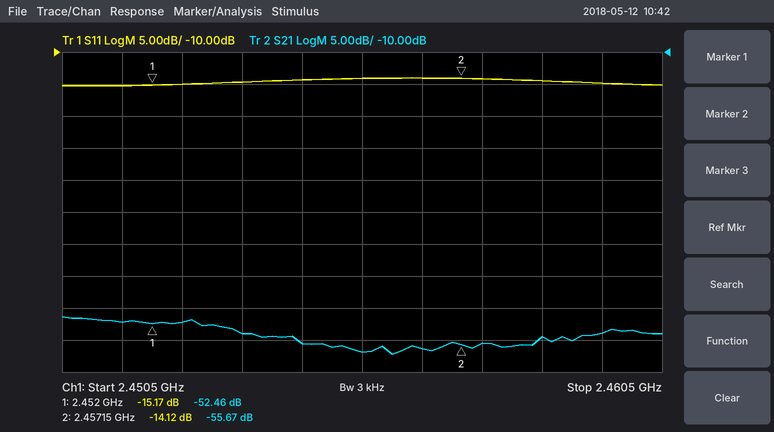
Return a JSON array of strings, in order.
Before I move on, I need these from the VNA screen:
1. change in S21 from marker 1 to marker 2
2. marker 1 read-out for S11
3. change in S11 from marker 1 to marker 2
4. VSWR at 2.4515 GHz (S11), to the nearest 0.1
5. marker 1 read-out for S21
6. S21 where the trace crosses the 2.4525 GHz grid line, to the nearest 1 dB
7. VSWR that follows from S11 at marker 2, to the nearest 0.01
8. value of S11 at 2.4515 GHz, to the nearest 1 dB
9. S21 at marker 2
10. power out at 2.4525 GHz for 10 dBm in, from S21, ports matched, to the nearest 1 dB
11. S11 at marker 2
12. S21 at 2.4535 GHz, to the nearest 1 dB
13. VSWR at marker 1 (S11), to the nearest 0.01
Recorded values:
["-3.21 dB", "-15.17 dB", "1.05 dB", "1.4", "-52.46 dB", "-52 dB", "1.49", "-15 dB", "-55.67 dB", "-42 dBm", "-14.12 dB", "-54 dB", "1.42"]
